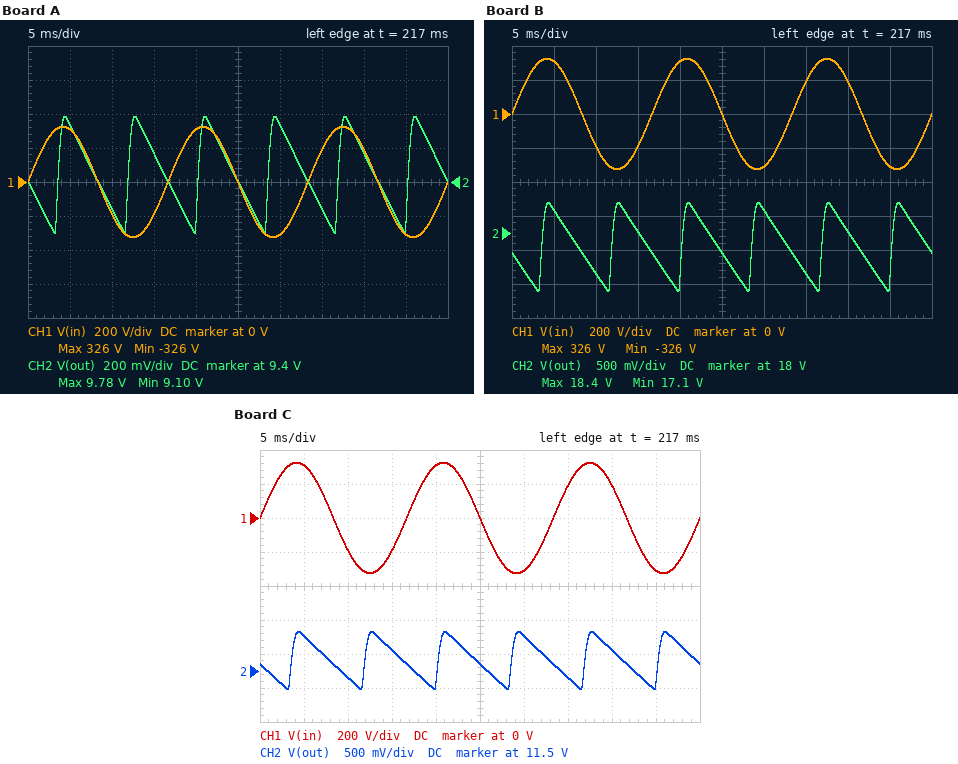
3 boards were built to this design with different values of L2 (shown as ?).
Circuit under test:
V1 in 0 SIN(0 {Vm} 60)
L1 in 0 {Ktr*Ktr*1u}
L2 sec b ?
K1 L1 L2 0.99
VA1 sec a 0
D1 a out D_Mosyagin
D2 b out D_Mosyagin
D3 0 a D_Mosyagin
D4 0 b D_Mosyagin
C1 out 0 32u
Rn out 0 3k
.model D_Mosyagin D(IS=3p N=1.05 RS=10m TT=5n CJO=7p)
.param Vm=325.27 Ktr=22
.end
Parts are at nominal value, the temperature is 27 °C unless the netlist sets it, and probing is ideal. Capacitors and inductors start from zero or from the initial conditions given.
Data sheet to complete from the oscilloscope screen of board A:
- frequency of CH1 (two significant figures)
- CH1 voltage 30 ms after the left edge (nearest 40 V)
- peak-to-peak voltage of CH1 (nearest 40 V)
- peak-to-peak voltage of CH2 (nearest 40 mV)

60 Hz
-320 V
640 V
680 mV
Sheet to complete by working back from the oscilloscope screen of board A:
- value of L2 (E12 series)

560 nH
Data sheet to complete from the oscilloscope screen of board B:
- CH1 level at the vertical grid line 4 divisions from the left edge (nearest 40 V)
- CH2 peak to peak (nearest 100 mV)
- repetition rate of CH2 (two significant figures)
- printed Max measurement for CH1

320 V
1.3 V
120 Hz
326 V
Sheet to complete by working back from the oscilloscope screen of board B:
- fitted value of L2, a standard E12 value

1.8 µH
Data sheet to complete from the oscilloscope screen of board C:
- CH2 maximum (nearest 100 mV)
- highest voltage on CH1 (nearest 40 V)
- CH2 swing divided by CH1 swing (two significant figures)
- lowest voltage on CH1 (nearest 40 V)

12.1 V
320 V
0.0013
-320 V
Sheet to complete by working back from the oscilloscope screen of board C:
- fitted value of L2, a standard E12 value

820 nH
